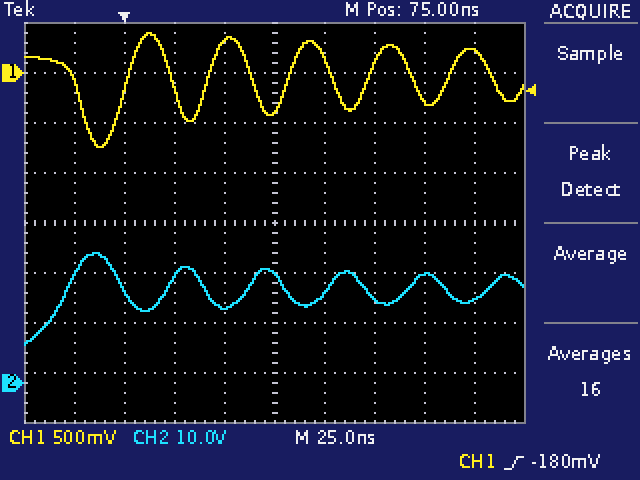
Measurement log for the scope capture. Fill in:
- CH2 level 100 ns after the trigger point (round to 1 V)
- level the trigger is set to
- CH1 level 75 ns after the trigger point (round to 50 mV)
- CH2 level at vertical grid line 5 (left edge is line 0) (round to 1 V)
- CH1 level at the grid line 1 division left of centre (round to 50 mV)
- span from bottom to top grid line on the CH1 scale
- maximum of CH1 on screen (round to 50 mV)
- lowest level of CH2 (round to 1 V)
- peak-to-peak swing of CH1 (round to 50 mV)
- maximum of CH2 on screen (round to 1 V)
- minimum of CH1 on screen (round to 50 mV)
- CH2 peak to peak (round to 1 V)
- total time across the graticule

18 V
-180 mV
-400 mV
22 V
300 mV
4 V
400 mV
8 V
1.15 V
26 V
-750 mV
18 V
250 ns
